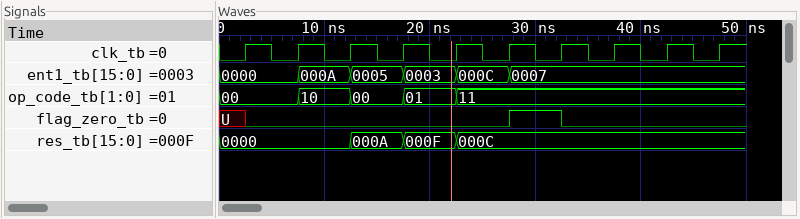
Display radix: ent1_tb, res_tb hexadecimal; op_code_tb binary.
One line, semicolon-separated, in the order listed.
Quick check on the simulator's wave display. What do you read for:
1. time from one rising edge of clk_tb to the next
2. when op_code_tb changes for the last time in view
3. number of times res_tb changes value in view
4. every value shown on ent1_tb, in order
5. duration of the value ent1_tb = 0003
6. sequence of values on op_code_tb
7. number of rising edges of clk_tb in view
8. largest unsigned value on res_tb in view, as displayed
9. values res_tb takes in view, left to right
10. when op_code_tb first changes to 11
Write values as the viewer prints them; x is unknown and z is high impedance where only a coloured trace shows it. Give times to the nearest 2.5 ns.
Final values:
5 ns; 22.5 ns; 3; 0000, 000A, 0005, 0003, 000C, 0007; 5 ns; 00, 10, 00, 01, 11; 10; 000F; 0000, 000A, 000F, 000C; 22.5 ns
